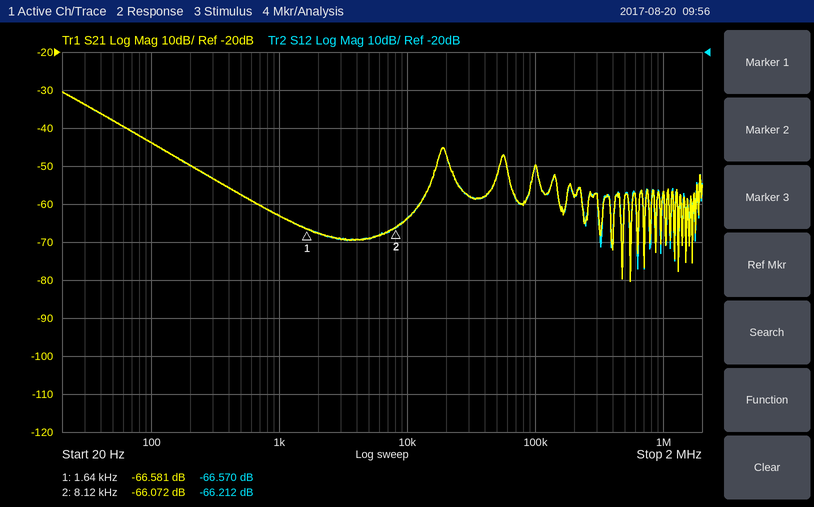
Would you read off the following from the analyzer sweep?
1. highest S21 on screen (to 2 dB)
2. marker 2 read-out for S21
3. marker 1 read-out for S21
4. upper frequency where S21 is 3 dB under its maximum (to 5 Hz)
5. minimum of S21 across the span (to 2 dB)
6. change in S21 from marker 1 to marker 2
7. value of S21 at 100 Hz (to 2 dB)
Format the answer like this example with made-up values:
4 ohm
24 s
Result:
-30 dB
-66.072 dB
-66.581 dB
30 Hz
-80 dB
0.509 dB
-44 dB
